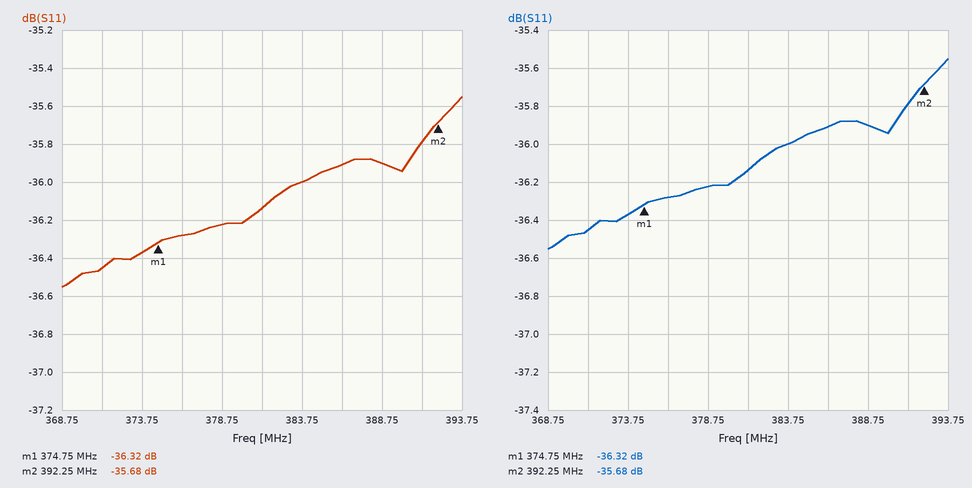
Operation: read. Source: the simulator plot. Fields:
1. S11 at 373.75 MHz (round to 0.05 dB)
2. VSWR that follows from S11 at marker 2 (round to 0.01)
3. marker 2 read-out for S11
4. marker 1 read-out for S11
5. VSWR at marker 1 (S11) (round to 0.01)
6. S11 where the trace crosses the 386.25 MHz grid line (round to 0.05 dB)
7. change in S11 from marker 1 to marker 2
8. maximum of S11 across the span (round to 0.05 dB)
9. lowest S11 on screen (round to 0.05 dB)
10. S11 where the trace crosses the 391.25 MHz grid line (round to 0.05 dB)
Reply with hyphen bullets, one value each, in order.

- -36.35 dB
- 1.03
- -35.68 dB
- -36.32 dB
- 1.03
- -35.90 dB
- 0.64 dB
- -35.55 dB
- -36.55 dB
- -35.80 dB
